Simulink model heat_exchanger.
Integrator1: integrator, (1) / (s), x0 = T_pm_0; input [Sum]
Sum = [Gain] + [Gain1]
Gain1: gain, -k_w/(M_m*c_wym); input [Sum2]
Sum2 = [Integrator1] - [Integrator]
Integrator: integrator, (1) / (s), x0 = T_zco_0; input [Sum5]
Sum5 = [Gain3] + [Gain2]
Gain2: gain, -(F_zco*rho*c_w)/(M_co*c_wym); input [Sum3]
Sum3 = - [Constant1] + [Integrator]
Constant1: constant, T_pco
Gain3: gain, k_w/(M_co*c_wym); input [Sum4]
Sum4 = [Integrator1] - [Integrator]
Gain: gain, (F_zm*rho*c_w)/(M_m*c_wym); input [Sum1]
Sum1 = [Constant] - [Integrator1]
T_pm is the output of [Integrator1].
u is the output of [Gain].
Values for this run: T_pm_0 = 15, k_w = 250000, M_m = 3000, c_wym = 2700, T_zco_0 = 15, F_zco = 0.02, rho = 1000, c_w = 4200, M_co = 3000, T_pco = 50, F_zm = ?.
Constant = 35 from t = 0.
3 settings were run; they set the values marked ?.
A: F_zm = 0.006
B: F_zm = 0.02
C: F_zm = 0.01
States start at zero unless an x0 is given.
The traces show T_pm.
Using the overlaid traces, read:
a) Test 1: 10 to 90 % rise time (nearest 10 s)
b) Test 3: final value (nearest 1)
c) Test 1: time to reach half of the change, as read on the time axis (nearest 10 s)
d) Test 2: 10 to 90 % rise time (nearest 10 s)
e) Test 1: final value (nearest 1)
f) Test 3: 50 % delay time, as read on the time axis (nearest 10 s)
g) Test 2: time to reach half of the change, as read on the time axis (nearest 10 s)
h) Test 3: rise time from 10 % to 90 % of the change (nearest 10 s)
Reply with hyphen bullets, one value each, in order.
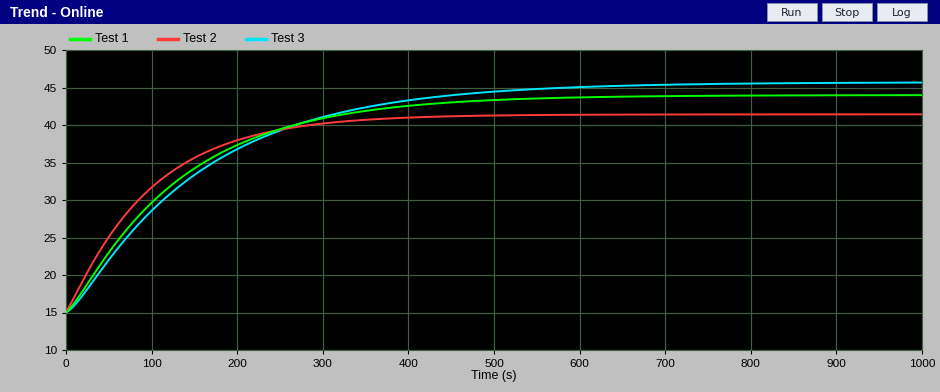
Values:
- 290 s
- 46
- 100 s
- 210 s
- 44
- 120 s
- 70 s
- 340 s
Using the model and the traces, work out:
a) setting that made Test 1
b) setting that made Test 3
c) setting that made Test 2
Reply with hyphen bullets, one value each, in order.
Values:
- C
- A
- B
